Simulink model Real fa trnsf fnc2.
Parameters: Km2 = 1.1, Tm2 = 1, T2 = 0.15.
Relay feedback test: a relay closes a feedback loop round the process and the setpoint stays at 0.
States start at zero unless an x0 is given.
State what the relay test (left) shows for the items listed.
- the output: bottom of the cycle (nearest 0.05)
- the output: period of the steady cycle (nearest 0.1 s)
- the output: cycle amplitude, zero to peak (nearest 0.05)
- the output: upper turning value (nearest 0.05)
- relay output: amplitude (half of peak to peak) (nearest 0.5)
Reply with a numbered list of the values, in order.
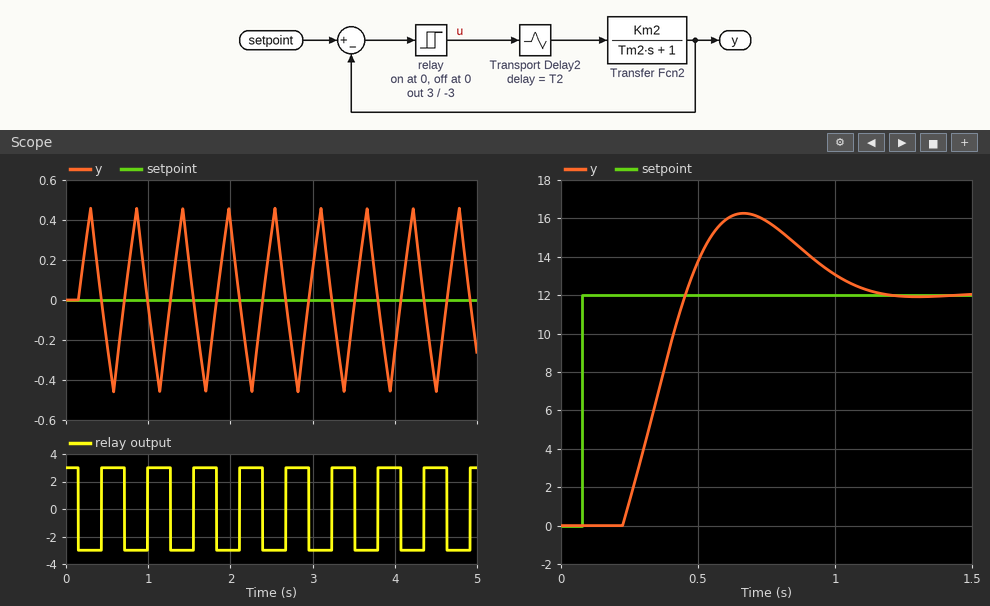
1. -0.45
2. 0.6 s
3. 0.45
4. 0.45
5. 3.0
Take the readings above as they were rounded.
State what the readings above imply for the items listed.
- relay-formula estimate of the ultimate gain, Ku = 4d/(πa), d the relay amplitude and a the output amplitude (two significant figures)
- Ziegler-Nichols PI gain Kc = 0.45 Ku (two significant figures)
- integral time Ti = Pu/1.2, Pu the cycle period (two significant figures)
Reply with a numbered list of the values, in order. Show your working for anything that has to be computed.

1. 4 × 3 / (π × 0.45) = 8.5
2. 0.45 × 8.5 = 3.8
3. 0.6 / 1.2 = 0.50 s
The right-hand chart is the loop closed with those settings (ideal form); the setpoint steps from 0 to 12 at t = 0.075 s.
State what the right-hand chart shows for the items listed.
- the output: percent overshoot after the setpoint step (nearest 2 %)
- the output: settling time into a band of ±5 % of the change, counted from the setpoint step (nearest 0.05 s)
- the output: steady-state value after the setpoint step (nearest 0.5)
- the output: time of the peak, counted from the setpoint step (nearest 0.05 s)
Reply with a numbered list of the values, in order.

1. 36 %
2. 1.00 s
3. 12.0
4. 0.60 s
